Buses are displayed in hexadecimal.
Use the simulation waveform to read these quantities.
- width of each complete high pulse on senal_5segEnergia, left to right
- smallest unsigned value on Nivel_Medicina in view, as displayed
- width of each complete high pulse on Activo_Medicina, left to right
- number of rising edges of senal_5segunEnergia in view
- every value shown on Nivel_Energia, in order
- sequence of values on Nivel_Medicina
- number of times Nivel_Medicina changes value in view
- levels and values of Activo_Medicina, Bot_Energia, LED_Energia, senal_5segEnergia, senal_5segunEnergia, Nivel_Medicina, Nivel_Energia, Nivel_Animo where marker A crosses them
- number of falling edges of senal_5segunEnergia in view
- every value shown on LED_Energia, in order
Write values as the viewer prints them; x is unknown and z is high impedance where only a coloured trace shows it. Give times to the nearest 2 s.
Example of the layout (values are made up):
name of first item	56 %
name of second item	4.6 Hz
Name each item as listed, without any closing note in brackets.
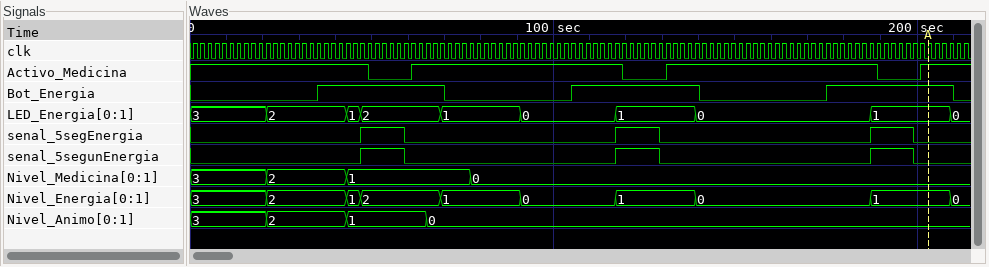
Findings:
width of each complete high pulse on senal_5segEnergia, left to right	12 s, 12 s, 12 s
smallest unsigned value on Nivel_Medicina in view, as displayed	0
width of each complete high pulse on Activo_Medicina, left to right	58 s, 58 s
number of rising edges of senal_5segunEnergia in view	3
every value shown on Nivel_Energia, in order	3, 2, 1, 2, 1, 0, 1, 0, 1, 0
sequence of values on Nivel_Medicina	3, 2, 1, 0
number of times Nivel_Medicina changes value in view	3
levels and values of Activo_Medicina, Bot_Energia, LED_Energia, senal_5segEnergia, senal_5segunEnergia, Nivel_Medicina, Nivel_Energia, Nivel_Animo where marker A crosses them	Activo_Medicina=1, Bot_Energia=1, LED_Energia=1, senal_5segEnergia=0, senal_5segunEnergia=0, Nivel_Medicina=0, Nivel_Energia=1, Nivel_Animo=0
number of falling edges of senal_5segunEnergia in view	3
every value shown on LED_Energia, in order	3, 2, 1, 2, 1, 0, 1, 0, 1, 0
